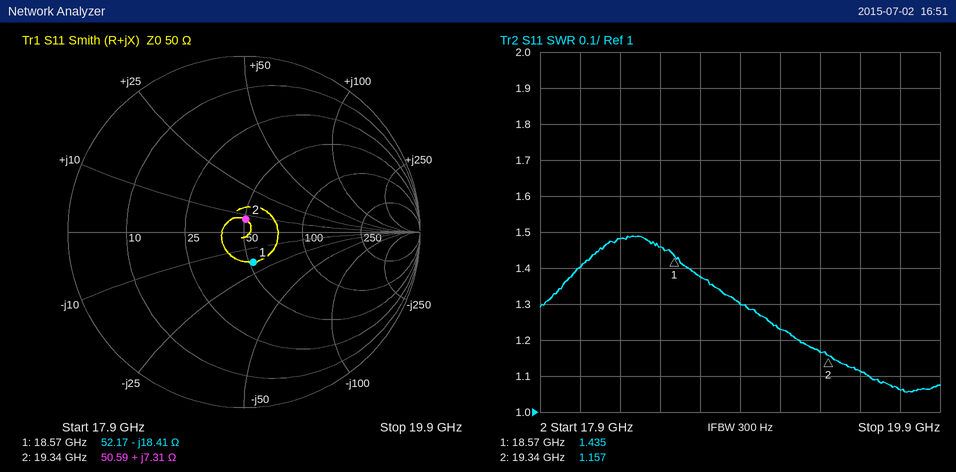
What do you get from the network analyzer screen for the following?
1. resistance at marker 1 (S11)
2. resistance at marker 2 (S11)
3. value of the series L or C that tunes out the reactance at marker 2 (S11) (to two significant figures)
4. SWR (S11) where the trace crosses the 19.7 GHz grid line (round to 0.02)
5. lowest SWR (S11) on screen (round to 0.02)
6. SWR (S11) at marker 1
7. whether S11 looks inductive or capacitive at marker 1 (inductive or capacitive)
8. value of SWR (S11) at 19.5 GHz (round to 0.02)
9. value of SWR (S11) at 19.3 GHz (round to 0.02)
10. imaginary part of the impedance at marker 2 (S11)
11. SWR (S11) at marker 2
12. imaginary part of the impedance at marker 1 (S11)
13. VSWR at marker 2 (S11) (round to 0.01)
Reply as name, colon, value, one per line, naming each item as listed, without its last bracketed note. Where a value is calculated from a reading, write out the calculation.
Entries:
resistance at marker 1: 52.17 Ω
resistance at marker 2: 50.59 Ω
value of the series L or C that tunes out the reactance at marker 2 (S11): C = 1/(2π × 19.34 GHz × 7.31 Ω) ≈ 1.1 pF
SWR (S11) where the trace crosses the 19.7 GHz grid line: 1.06
lowest SWR (S11) on screen: 1.06
SWR (S11) at marker 1: 1.435
whether S11 looks inductive or capacitive at marker 1: capacitive
value of SWR (S11) at 19.5 GHz: 1.12
value of SWR (S11) at 19.3 GHz: 1.16
imaginary part of the impedance at marker 2: +7.31 Ω
SWR (S11) at marker 2: 1.157
imaginary part of the impedance at marker 1: -18.41 Ω
VSWR at marker 2 (S11): 1.16
